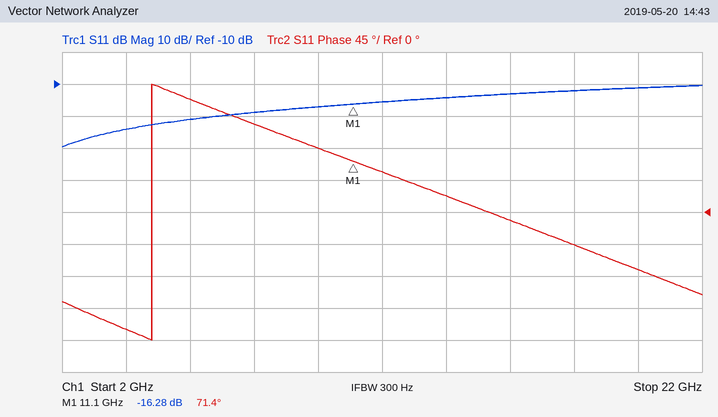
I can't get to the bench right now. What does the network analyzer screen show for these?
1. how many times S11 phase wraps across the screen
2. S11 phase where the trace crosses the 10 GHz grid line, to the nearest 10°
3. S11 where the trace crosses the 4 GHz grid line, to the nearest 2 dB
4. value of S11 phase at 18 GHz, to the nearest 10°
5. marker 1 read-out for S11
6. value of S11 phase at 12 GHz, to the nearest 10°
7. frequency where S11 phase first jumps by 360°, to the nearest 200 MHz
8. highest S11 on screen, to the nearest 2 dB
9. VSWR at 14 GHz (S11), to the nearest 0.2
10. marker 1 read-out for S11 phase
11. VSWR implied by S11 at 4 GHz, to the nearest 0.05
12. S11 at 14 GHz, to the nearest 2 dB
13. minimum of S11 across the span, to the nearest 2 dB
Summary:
1
90°
-24 dB
-50°
-16.28 dB
60°
4.8 GHz
-10 dB
1.4
71.4°
1.15
-14 dB
-30 dB
